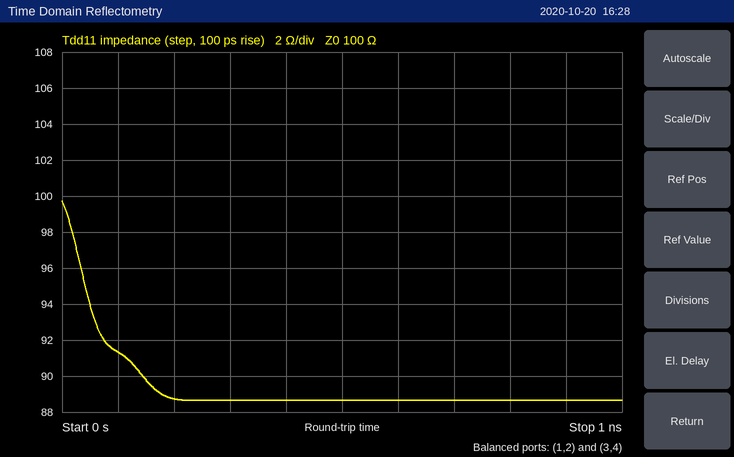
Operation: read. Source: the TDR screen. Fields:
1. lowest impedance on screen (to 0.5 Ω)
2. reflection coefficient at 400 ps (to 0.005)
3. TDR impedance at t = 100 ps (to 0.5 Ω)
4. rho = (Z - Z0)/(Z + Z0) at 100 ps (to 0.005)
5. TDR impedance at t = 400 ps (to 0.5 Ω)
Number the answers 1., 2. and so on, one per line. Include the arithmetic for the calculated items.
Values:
1. 88.5 Ω
2. (88.5 − 100)/(88.5 + 100) ≈ -0.0610, so -0.060 to the nearest 0.005
3. 91.5 Ω
4. (91.5 − 100)/(91.5 + 100) ≈ -0.0444, so -0.045 to the nearest 0.005
5. 88.5 Ω
